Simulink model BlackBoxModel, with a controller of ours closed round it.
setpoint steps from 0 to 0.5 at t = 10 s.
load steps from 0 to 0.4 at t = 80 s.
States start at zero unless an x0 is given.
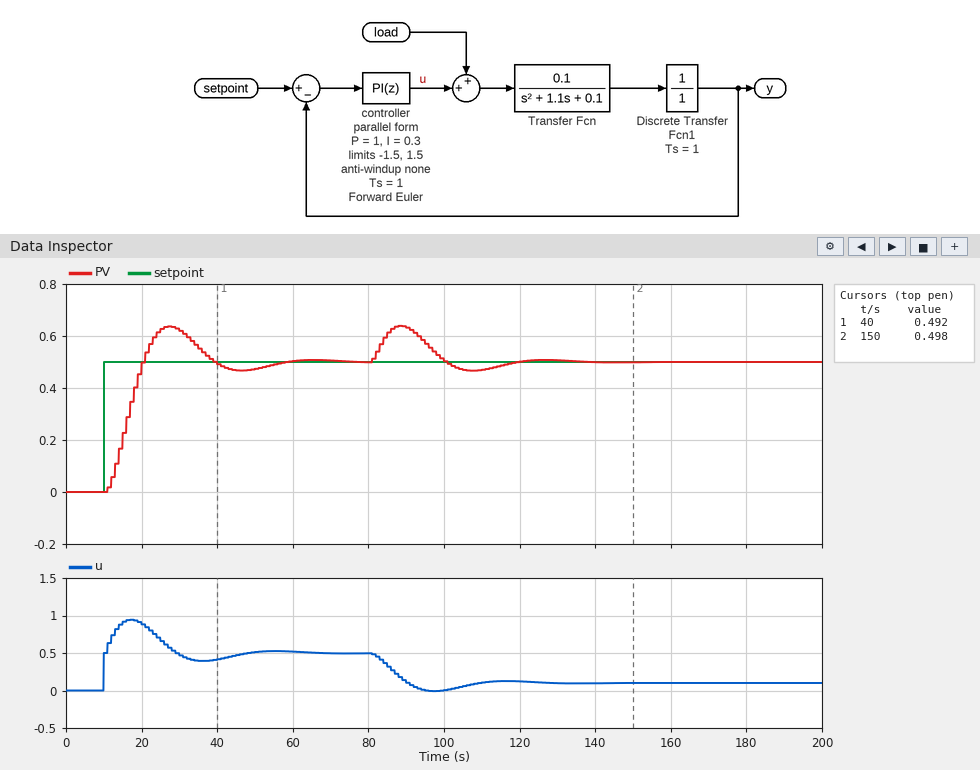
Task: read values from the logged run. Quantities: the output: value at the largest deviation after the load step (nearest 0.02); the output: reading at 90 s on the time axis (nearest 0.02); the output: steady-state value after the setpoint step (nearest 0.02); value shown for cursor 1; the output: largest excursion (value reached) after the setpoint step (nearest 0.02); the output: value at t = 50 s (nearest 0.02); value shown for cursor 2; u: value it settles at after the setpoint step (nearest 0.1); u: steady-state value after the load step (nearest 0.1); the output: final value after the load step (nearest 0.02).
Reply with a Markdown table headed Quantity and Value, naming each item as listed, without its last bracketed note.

| Quantity | Value |
|---|---|
| the output: value at the largest deviation after the load step | 0.64 |
| the output: reading at 90 s on the time axis | 0.64 |
| the output: steady-state value after the setpoint step | 0.50 |
| value shown for cursor 1 | 0.492 |
| the output: largest excursion (value reached) after the setpoint step | 0.64 |
| the output: value at t = 50 s | 0.48 |
| value shown for cursor 2 | 0.498 |
| u: value it settles at after the setpoint step | 0.5 |
| u: steady-state value after the load step | 0.1 |
| the output: final value after the load step | 0.50 |
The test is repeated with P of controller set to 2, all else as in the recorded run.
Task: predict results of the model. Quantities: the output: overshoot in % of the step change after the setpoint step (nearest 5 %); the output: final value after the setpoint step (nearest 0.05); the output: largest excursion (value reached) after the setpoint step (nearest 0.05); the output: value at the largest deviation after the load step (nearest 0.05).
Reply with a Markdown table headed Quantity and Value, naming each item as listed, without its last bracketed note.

| Quantity | Value |
|---|---|
| the output: overshoot in % of the step change after the setpoint step | 10 % |
| the output: final value after the setpoint step | 0.50 |
| the output: largest excursion (value reached) after the setpoint step | 0.55 |
| the output: value at the largest deviation after the load step | 0.60 |
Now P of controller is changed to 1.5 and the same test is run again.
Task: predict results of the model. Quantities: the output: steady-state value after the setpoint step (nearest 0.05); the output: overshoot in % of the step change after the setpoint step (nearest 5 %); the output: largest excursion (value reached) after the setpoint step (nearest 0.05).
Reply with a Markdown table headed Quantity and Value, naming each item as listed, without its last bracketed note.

| Quantity | Value |
|---|---|
| the output: steady-state value after the setpoint step | 0.50 |
| the output: overshoot in % of the step change after the setpoint step | 15 % |
| the output: largest excursion (value reached) after the setpoint step | 0.60 |
